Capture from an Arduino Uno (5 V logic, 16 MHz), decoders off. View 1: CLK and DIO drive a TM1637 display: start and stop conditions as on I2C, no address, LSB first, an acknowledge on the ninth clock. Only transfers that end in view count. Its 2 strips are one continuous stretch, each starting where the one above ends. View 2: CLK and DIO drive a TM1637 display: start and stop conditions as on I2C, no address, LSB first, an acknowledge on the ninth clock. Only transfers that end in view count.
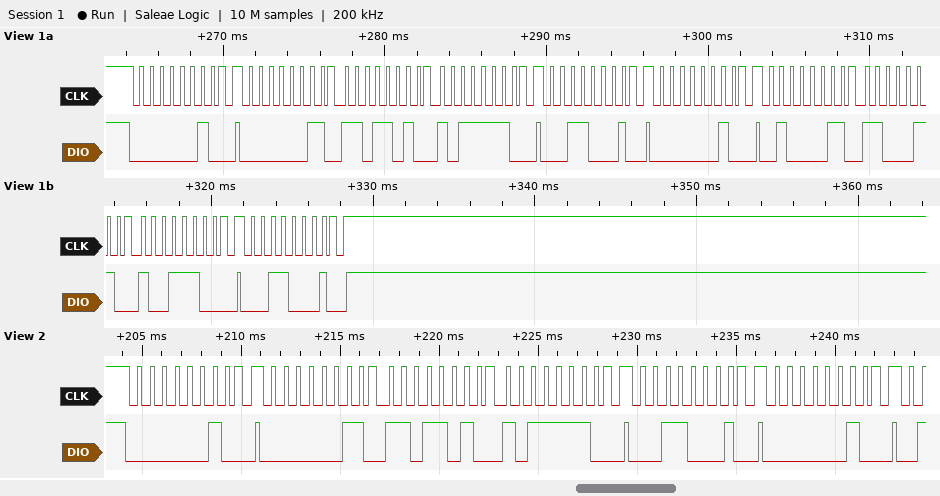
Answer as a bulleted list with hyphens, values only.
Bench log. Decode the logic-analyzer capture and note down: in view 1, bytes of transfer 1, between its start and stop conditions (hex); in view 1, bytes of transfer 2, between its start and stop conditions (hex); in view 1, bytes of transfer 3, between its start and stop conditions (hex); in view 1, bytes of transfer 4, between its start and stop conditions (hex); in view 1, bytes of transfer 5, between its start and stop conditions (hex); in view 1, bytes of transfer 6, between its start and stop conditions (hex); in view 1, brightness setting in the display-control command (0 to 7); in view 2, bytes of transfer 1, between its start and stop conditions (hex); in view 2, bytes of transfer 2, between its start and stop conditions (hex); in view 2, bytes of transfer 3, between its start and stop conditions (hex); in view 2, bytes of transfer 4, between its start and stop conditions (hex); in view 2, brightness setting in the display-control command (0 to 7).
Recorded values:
- 40
- C0 5B 7D
- 8C
- 40
- C2 63 39
- 8C
- 4
- 40
- C0 5B 7D
- 8C
- 40
- 4
